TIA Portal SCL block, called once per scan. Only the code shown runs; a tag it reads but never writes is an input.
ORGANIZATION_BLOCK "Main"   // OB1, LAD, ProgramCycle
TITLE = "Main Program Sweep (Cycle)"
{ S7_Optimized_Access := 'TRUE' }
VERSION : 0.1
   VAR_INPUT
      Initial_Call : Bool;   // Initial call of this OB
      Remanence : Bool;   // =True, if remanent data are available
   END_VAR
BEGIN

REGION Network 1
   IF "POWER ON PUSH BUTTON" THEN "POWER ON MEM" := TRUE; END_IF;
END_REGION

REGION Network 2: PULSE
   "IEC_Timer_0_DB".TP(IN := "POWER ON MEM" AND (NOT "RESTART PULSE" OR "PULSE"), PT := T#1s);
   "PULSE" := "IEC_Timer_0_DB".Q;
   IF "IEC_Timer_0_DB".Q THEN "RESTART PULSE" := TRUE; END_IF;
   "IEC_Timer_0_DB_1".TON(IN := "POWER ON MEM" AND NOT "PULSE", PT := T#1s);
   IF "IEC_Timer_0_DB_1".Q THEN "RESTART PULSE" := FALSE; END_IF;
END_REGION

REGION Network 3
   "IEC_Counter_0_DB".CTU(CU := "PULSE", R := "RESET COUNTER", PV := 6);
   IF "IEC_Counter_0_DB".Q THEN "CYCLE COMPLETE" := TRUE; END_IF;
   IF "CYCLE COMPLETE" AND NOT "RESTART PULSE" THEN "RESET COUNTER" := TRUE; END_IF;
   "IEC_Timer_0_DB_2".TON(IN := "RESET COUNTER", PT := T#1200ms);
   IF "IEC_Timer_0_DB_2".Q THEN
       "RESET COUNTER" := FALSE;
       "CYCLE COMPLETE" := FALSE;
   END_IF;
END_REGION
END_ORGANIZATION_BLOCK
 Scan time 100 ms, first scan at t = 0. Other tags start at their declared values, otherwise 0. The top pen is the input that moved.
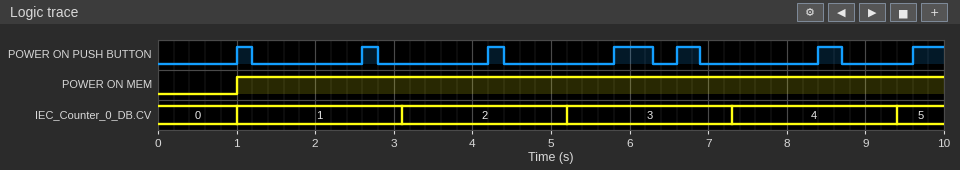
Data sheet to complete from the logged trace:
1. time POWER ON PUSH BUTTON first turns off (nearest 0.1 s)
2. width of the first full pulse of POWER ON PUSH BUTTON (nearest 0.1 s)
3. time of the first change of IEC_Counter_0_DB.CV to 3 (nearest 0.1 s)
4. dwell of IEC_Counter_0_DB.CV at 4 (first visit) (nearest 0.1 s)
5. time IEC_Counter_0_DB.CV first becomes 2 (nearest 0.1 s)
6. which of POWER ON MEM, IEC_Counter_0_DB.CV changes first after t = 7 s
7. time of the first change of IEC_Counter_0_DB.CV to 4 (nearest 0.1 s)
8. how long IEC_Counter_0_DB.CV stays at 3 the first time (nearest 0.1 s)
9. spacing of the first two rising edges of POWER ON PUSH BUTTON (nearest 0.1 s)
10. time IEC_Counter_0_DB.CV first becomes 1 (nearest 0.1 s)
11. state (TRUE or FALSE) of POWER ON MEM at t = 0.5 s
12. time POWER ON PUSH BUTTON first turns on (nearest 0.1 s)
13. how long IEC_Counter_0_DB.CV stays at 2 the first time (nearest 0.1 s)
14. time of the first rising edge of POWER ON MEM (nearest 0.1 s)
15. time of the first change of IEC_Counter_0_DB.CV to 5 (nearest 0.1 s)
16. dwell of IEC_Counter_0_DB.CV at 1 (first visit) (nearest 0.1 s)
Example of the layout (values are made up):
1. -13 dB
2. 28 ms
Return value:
1. 1.2 s
2. 0.2 s
3. 5.2 s
4. 2.1 s
5. 3.1 s
6. IEC_Counter_0_DB.CV
7. 7.3 s
8. 2.1 s
9. 1.6 s
10. 1.0 s
11. FALSE
12. 1.0 s
13. 2.1 s
14. 1.0 s
15. 9.4 s
16. 2.1 s
